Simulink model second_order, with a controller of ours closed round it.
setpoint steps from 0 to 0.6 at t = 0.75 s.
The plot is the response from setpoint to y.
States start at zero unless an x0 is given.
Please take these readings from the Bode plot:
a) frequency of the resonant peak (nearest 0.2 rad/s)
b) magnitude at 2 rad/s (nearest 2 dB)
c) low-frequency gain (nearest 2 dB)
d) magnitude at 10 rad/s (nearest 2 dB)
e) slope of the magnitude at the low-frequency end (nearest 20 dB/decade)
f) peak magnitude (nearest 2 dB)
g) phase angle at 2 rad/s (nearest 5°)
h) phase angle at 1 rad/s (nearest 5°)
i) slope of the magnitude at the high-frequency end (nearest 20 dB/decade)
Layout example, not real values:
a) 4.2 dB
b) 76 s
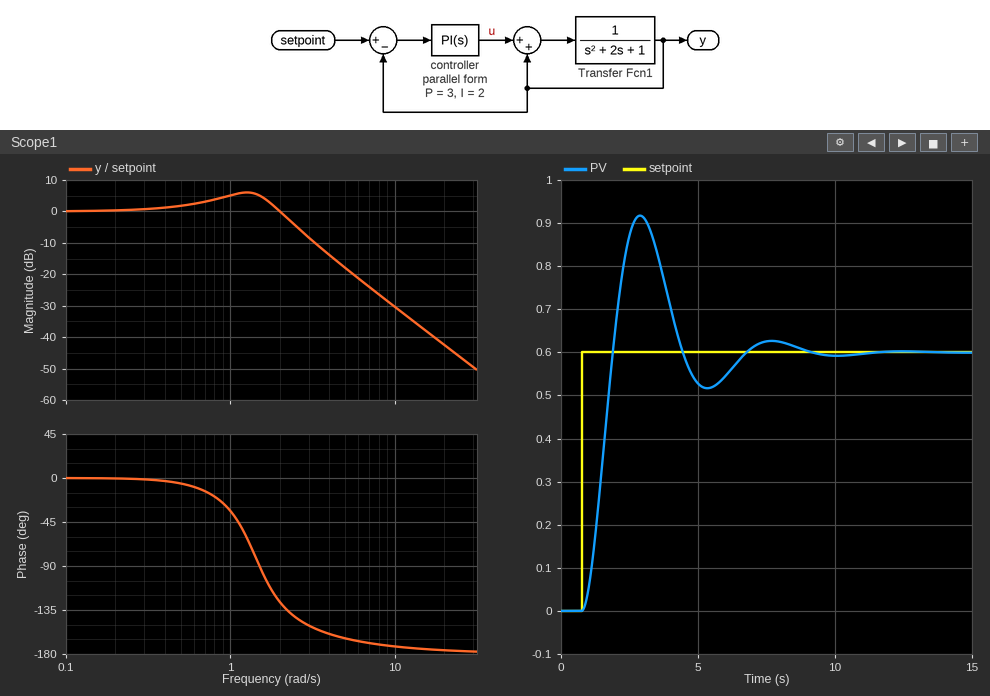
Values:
a) 1.2 rad/s
b) 0 dB
c) 0 dB
d) -30 dB
e) 0 dB/decade
f) 6 dB
g) -125°
h) -35°
i) -40 dB/decade
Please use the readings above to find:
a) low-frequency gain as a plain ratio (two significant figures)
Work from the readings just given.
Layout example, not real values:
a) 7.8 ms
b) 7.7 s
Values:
a) 1.0
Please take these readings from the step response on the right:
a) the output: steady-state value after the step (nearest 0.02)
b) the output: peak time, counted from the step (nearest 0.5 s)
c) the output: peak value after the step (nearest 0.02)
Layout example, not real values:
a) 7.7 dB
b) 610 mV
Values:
a) 0.60
b) 2.0 s
c) 0.92
